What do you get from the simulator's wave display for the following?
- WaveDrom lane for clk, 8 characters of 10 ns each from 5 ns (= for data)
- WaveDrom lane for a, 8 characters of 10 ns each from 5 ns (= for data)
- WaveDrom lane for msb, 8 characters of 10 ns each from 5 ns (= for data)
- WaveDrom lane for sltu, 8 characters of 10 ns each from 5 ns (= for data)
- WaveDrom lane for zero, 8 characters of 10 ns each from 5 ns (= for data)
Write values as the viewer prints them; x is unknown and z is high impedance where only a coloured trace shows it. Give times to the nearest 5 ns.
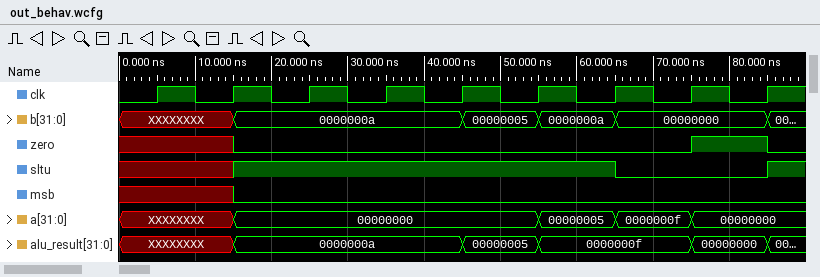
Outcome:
{name: 'clk', wave: 'p.......'}
{name: 'a', wave: 'x=...===', data: '00000000 00000005 0000000f 00000000'}
{name: 'msb', wave: 'x0......'}
{name: 'sltu', wave: 'x1....0.'}
{name: 'zero', wave: 'x0.....1'}
